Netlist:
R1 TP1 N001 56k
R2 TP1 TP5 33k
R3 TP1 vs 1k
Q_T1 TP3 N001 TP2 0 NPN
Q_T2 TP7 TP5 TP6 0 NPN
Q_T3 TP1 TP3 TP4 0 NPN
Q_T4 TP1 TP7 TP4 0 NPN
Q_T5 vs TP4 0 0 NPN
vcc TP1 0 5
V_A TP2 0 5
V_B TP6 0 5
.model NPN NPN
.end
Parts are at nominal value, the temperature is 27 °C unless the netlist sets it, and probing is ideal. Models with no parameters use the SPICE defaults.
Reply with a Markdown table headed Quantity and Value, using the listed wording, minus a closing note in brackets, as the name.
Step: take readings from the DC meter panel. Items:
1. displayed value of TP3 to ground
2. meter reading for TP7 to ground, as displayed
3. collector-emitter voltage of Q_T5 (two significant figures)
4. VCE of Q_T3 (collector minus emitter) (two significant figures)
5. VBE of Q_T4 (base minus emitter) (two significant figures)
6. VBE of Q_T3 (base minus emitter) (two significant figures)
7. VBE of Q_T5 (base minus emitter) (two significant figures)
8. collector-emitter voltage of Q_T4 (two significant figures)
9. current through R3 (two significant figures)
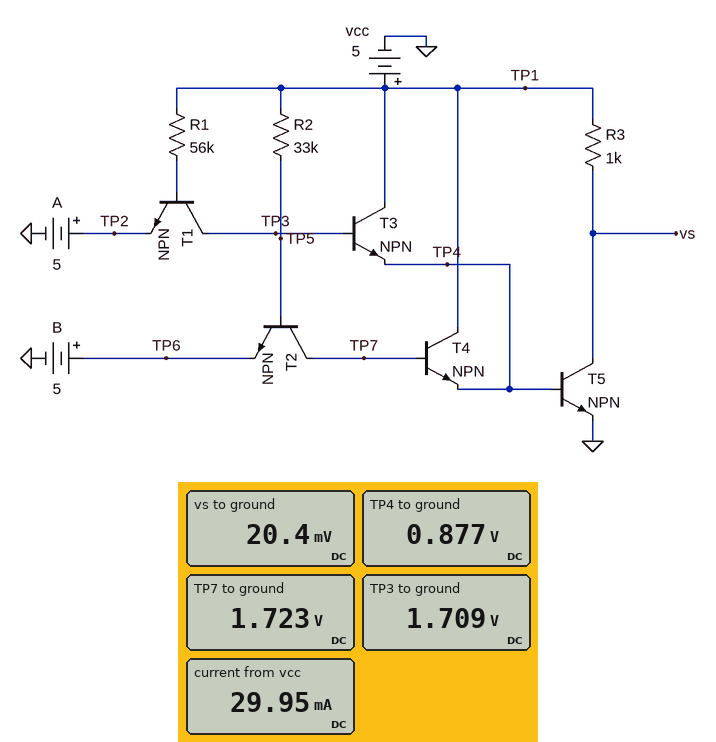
| Quantity | Value |
|---|---|
| displayed value of TP3 to ground | 1.709 V |
| meter reading for TP7 to ground, as displayed | 1.723 V |
| collector-emitter voltage of Q_T5 | 20 mV |
| VCE of Q_T3 (collector minus emitter) | 4.1 V |
| VBE of Q_T4 (base minus emitter) | 850 mV |
| VBE of Q_T3 (base minus emitter) | 830 mV |
| VBE of Q_T5 (base minus emitter) | 880 mV |
| collector-emitter voltage of Q_T4 | 4.1 V |
| current through R3 | 5.0 mA |
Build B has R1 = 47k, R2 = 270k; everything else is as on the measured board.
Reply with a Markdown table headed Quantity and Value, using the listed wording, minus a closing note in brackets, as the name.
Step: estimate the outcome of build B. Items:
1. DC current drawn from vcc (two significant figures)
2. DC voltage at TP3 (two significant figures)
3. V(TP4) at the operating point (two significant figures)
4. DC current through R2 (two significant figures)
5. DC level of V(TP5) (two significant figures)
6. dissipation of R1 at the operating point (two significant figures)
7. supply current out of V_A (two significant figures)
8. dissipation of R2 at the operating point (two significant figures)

| Quantity | Value |
|---|---|
| DC current drawn from vcc | 18 mA |
| DC voltage at TP3 | 1.7 V |
| V(TP4) at the operating point | 860 mV |
| DC current through R2 | 10 µA |
| DC level of V(TP5) | 2.3 V |
| dissipation of R1 at the operating point | 140 µW |
| supply current out of V_A | 55 µA |
| dissipation of R2 at the operating point | 27 µW |
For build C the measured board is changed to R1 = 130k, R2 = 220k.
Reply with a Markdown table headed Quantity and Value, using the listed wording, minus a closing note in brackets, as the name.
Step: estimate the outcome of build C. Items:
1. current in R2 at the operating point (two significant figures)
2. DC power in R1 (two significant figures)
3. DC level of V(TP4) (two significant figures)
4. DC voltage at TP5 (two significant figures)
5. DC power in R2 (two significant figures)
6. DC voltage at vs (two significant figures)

| Quantity | Value |
|---|---|
| current in R2 at the operating point | 12 µA |
| DC power in R1 | 55 µW |
| DC level of V(TP4) | 850 mV |
| DC voltage at TP5 | 2.3 V |
| DC power in R2 | 33 µW |
| DC voltage at vs | 26 mV |
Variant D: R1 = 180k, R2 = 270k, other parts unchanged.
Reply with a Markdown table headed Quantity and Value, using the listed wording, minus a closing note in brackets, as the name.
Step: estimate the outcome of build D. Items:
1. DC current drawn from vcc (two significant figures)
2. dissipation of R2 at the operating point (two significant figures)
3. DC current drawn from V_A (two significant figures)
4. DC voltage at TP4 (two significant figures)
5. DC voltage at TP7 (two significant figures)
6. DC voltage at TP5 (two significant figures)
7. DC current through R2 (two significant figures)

| Quantity | Value |
|---|---|
| DC current drawn from vcc | 10 mA |
| dissipation of R2 at the operating point | 27 µW |
| DC current drawn from V_A | 15 µA |
| DC voltage at TP4 | 840 mV |
| DC voltage at TP7 | 1.6 V |
| DC voltage at TP5 | 2.3 V |
| DC current through R2 | 10 µA |
